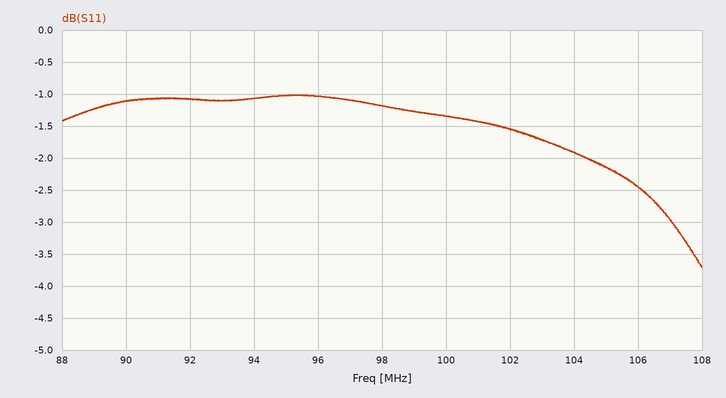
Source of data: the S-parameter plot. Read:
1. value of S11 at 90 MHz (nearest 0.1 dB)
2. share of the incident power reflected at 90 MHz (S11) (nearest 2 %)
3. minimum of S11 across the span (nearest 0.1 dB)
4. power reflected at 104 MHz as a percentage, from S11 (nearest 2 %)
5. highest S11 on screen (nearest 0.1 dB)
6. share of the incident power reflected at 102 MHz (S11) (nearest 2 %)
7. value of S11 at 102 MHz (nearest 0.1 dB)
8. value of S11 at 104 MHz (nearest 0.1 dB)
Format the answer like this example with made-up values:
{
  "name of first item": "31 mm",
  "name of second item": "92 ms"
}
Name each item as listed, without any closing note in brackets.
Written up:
{
  "value of S11 at 90 MHz": "-1.1 dB",
  "share of the incident power reflected at 90 MHz (S11)": "78 %",
  "minimum of S11 across the span": "-3.7 dB",
  "power reflected at 104 MHz as a percentage, from S11": "64 %",
  "highest S11 on screen": "-1.0 dB",
  "share of the incident power reflected at 102 MHz (S11)": "70 %",
  "value of S11 at 102 MHz": "-1.5 dB",
  "value of S11 at 104 MHz": "-1.9 dB"
}
